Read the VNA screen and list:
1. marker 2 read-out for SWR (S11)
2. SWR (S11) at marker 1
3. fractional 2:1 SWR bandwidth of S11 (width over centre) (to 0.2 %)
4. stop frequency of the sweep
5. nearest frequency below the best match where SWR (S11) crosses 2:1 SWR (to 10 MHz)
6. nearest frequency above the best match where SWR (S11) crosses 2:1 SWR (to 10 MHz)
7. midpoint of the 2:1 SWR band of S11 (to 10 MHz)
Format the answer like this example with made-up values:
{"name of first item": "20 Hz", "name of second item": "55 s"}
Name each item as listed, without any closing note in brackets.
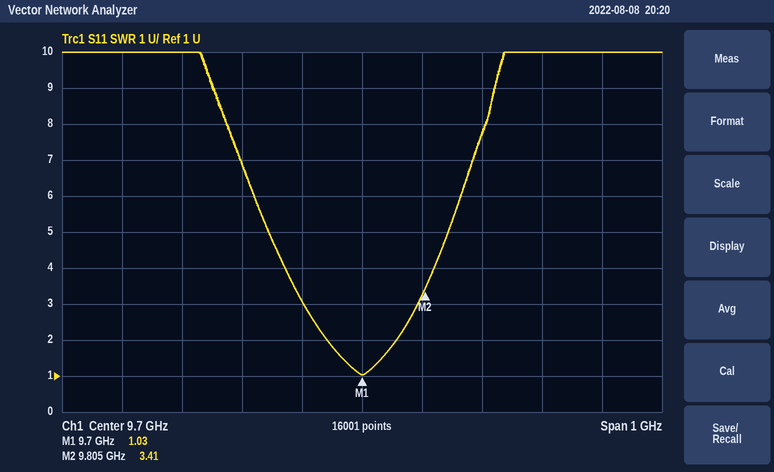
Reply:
{"marker 2 read-out for SWR": "3.41", "SWR (S11) at marker 1": "1.03", "fractional 2:1 SWR bandwidth of S11 (width over centre)": "1.2 %", "stop frequency of the sweep": "10.2 GHz", "nearest frequency below the best match where SWR (S11) crosses 2:1 SWR": "9.64 GHz", "nearest frequency above the best match where SWR (S11) crosses 2:1 SWR": "9.76 GHz", "midpoint of the 2:1 SWR band of S11": "9.70 GHz"}
